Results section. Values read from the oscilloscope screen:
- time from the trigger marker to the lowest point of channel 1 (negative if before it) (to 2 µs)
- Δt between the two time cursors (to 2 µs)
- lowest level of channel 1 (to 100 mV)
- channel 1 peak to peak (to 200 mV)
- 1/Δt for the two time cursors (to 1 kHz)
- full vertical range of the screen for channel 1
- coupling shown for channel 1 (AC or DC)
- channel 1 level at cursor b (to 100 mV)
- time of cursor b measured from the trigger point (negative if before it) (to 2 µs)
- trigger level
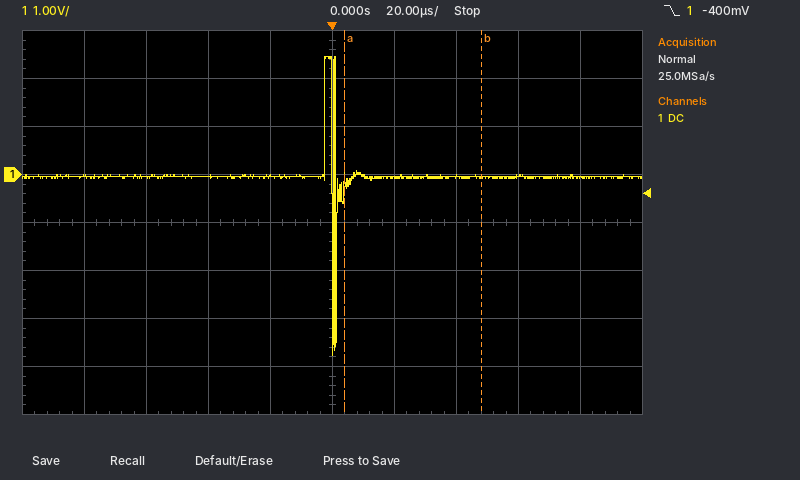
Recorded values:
0 µs
44 µs
-3.8 V
6.2 V
23 kHz
8 V
DC
-100 mV
+48 µs
-400 mV
